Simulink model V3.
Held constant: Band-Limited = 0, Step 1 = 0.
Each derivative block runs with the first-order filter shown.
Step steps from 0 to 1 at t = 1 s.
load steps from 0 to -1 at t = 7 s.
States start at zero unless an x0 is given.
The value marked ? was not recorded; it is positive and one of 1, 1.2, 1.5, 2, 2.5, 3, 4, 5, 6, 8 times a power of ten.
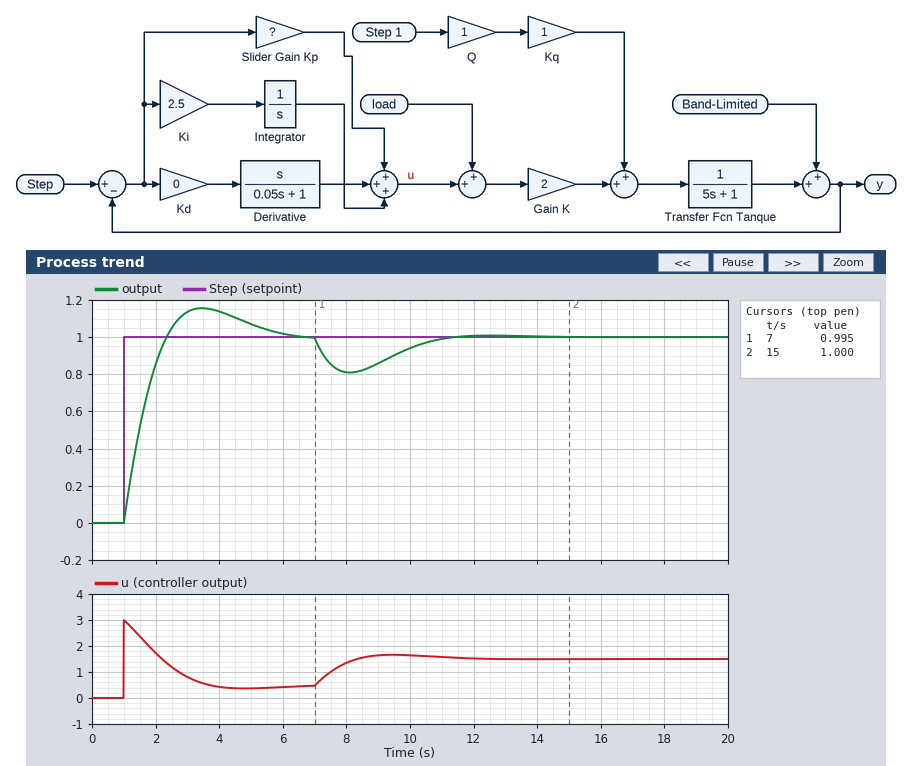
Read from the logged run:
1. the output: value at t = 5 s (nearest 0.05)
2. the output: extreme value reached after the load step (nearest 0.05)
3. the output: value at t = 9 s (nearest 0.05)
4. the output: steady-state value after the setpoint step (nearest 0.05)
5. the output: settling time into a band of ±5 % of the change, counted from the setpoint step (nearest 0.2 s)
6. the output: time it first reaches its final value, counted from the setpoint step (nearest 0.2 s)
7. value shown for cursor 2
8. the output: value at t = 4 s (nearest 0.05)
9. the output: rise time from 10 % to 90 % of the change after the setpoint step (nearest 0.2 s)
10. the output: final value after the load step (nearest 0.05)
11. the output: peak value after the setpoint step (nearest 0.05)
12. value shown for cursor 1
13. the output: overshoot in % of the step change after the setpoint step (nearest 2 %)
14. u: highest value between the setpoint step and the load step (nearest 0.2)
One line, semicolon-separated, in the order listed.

1.05; 0.80; 0.85; 1.00; 4.4 s; 1.4 s; 1.000; 1.15; 1.0 s; 1.00; 1.15; 0.995; 16 %; 3.0
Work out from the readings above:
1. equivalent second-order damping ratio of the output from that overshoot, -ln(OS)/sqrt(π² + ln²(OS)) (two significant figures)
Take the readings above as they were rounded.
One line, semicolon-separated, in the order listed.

0.50
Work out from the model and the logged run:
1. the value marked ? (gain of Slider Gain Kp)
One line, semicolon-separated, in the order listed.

3
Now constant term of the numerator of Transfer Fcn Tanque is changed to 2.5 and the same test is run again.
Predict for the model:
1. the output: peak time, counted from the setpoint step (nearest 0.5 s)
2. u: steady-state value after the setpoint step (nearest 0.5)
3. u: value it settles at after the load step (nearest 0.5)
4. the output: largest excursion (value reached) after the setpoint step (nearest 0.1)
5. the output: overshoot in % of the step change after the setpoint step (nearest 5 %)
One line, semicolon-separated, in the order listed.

1.5 s; 0.0; 1.0; 1.1; 10 %
